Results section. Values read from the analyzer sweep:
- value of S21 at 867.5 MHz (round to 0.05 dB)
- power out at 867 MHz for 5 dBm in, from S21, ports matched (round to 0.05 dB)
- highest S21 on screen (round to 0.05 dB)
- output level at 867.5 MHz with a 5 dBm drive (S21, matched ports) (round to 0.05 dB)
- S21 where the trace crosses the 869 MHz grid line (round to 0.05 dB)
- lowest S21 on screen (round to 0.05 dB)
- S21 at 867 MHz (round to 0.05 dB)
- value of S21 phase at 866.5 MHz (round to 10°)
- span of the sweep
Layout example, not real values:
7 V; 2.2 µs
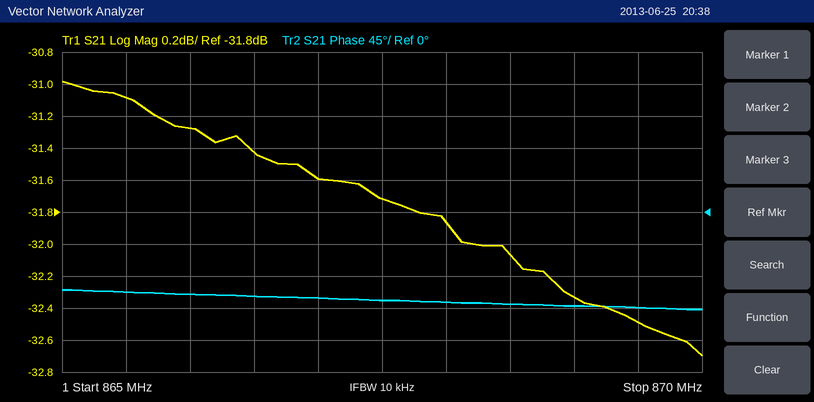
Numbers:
-31.70 dB; -26.60 dBm; -31.00 dB; -26.70 dBm; -32.35 dB; -32.70 dB; -31.60 dB; -120°; 5 MHz
